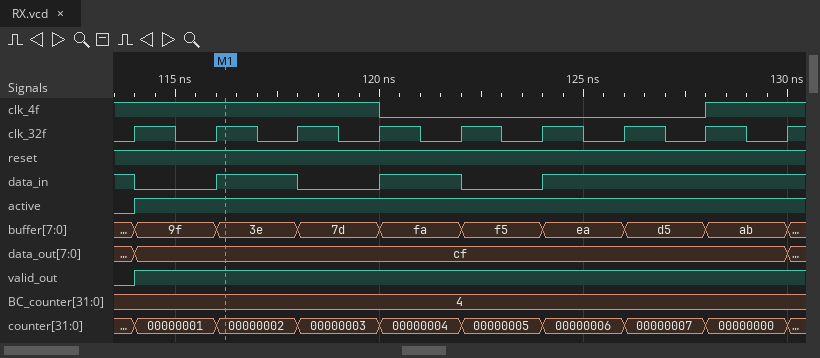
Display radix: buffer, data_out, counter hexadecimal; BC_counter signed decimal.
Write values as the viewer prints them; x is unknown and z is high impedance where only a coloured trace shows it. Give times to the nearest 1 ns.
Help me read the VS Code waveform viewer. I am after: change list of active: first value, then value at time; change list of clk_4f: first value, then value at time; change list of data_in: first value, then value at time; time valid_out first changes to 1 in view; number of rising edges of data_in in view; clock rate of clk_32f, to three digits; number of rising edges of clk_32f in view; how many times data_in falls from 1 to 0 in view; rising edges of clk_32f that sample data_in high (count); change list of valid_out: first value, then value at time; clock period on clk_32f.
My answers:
0, 1 at 114 ns
1, 0 at 120 ns, 1 at 128 ns
1, 0 at 114 ns, 1 at 116 ns, 0 at 118 ns, 1 at 120 ns, 0 at 122 ns, 1 at 124 ns
114 ns
3
500 MHz
9
3
6
0, 1 at 114 ns
2 ns
